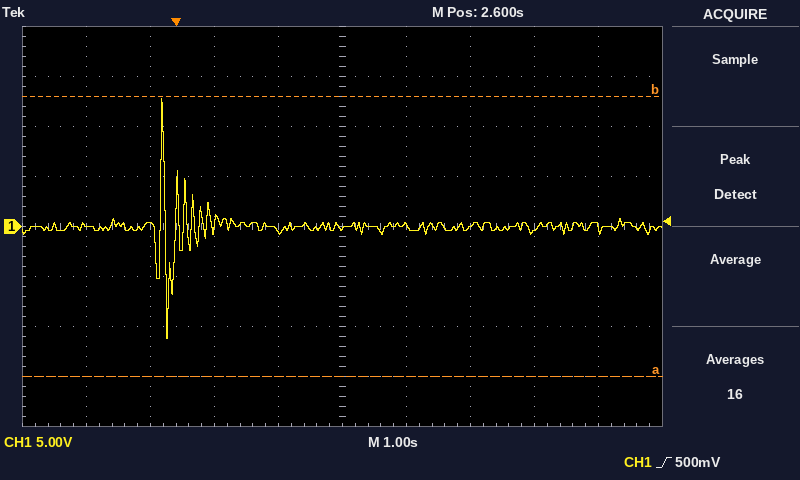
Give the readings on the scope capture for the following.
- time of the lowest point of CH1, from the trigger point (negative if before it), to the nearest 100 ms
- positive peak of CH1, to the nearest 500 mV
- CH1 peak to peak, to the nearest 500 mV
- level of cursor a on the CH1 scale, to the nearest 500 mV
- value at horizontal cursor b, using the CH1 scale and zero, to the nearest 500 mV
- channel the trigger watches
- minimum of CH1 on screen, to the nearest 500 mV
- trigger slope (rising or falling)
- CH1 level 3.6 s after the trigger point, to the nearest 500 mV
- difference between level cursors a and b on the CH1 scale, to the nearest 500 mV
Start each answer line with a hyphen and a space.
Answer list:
- -100 ms
- 13.0 V
- 24.0 V
- -15.0 V
- 13.0 V
- CH1
- -11.0 V
- rising
- 0.0 V
- 28.0 V
